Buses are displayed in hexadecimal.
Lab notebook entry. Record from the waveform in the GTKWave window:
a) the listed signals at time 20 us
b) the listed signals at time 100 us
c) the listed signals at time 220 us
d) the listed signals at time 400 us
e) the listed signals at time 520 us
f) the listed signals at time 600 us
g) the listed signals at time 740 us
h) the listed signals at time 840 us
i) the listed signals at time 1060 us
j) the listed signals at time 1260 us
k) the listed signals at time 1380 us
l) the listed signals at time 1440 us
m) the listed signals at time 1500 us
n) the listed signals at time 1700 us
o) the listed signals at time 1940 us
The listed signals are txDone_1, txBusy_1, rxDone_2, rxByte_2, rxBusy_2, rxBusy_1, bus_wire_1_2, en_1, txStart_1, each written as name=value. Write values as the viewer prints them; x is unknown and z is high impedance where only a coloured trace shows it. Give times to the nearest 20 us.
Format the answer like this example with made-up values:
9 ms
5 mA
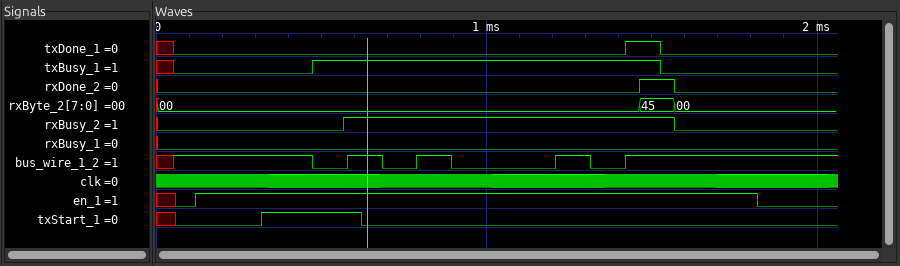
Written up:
txDone_1=x, txBusy_1=x, rxDone_2=0, rxByte_2=00, rxBusy_2=0, rxBusy_1=0, bus_wire_1_2=x, en_1=x, txStart_1=x
txDone_1=0, txBusy_1=0, rxDone_2=0, rxByte_2=00, rxBusy_2=0, rxBusy_1=0, bus_wire_1_2=1, en_1=0, txStart_1=0
txDone_1=0, txBusy_1=0, rxDone_2=0, rxByte_2=00, rxBusy_2=0, rxBusy_1=0, bus_wire_1_2=1, en_1=1, txStart_1=0
txDone_1=0, txBusy_1=0, rxDone_2=0, rxByte_2=00, rxBusy_2=0, rxBusy_1=0, bus_wire_1_2=1, en_1=1, txStart_1=1
txDone_1=0, txBusy_1=1, rxDone_2=0, rxByte_2=00, rxBusy_2=0, rxBusy_1=0, bus_wire_1_2=0, en_1=1, txStart_1=1
txDone_1=0, txBusy_1=1, rxDone_2=0, rxByte_2=00, rxBusy_2=1, rxBusy_1=0, bus_wire_1_2=1, en_1=1, txStart_1=1
txDone_1=0, txBusy_1=1, rxDone_2=0, rxByte_2=00, rxBusy_2=1, rxBusy_1=0, bus_wire_1_2=0, en_1=1, txStart_1=0
txDone_1=0, txBusy_1=1, rxDone_2=0, rxByte_2=00, rxBusy_2=1, rxBusy_1=0, bus_wire_1_2=1, en_1=1, txStart_1=0
txDone_1=0, txBusy_1=1, rxDone_2=0, rxByte_2=00, rxBusy_2=1, rxBusy_1=0, bus_wire_1_2=0, en_1=1, txStart_1=0
txDone_1=0, txBusy_1=1, rxDone_2=0, rxByte_2=00, rxBusy_2=1, rxBusy_1=0, bus_wire_1_2=1, en_1=1, txStart_1=0
txDone_1=0, txBusy_1=1, rxDone_2=0, rxByte_2=00, rxBusy_2=1, rxBusy_1=0, bus_wire_1_2=0, en_1=1, txStart_1=0
txDone_1=1, txBusy_1=1, rxDone_2=0, rxByte_2=00, rxBusy_2=1, rxBusy_1=0, bus_wire_1_2=1, en_1=1, txStart_1=0
txDone_1=1, txBusy_1=1, rxDone_2=1, rxByte_2=45, rxBusy_2=1, rxBusy_1=0, bus_wire_1_2=1, en_1=1, txStart_1=0
txDone_1=0, txBusy_1=0, rxDone_2=0, rxByte_2=00, rxBusy_2=0, rxBusy_1=0, bus_wire_1_2=1, en_1=1, txStart_1=0
txDone_1=0, txBusy_1=0, rxDone_2=0, rxByte_2=00, rxBusy_2=0, rxBusy_1=0, bus_wire_1_2=1, en_1=0, txStart_1=0
